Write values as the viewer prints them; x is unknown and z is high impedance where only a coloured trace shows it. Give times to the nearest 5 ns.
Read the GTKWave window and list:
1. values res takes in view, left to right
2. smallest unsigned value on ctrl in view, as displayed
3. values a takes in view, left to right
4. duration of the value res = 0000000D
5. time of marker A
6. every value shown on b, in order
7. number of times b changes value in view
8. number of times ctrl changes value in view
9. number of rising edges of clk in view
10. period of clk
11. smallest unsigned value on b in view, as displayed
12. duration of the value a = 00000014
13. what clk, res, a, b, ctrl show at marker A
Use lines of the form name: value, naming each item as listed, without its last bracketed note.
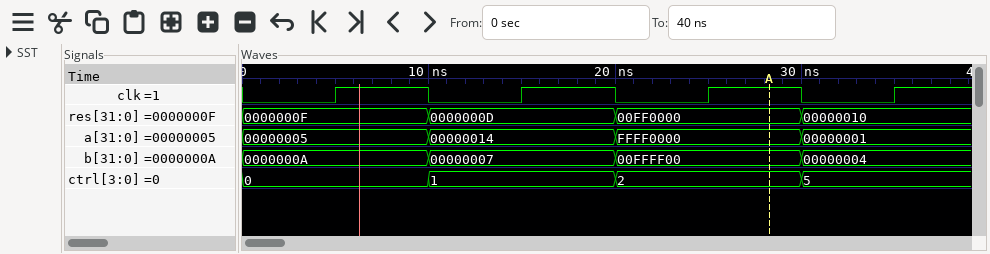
values res takes in view, left to right: 0000000F, 0000000D, 00FF0000, 00000010
smallest unsigned value on ctrl in view, as displayed: 0
values a takes in view, left to right: 00000005, 00000014, FFFF0000, 00000001
duration of the value res = 0000000D: 10 ns
time of marker A: 30 ns
every value shown on b, in order: 0000000A, 00000007, 00FFFF00, 00000004
number of times b changes value in view: 3
number of times ctrl changes value in view: 3
number of rising edges of clk in view: 4
period of clk: 10 ns
smallest unsigned value on b in view, as displayed: 00000004
duration of the value a = 00000014: 10 ns
what clk, res, a, b, ctrl show at marker A: clk=1, res=00FF0000, a=FFFF0000, b=00FFFF00, ctrl=2
